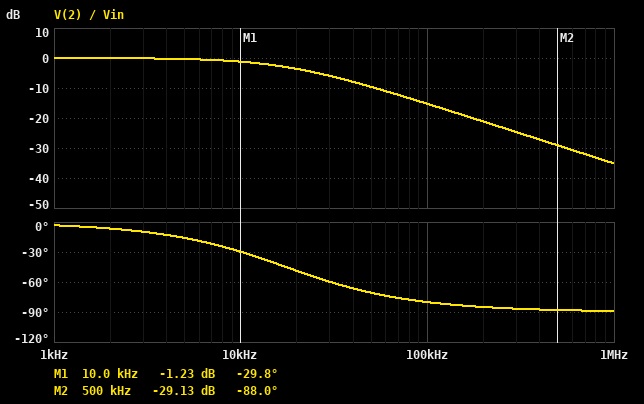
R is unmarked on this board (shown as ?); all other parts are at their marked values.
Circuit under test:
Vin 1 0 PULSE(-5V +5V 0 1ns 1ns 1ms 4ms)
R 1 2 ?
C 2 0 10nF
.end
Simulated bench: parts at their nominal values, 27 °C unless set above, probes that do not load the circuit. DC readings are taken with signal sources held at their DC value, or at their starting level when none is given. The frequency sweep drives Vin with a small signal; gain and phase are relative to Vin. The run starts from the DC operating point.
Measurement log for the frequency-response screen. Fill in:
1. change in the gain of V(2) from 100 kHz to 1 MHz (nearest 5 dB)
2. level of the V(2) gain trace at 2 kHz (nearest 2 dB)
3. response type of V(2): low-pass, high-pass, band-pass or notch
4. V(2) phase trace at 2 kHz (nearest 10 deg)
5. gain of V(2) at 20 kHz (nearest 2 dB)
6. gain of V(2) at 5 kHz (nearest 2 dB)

-20 dB
0 dB
low-pass
-10 deg
-4 dB
0 dB
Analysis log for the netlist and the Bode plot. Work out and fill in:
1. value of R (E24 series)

910 Ω
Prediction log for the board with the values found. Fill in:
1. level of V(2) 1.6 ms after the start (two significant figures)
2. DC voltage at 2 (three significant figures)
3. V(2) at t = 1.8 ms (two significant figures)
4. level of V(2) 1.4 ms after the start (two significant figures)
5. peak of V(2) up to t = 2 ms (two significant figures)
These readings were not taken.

-5.0 V
-5.00 V
-5.0 V
-5.0 V
5.0 V
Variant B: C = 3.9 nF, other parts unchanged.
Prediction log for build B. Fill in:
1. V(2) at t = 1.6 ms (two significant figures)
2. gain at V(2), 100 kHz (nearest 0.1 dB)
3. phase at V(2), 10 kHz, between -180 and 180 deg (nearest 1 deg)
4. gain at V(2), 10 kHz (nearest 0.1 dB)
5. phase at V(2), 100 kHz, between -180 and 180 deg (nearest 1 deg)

-5.0 V
-7.8 dB
-13 deg
-0.2 dB
-66 deg
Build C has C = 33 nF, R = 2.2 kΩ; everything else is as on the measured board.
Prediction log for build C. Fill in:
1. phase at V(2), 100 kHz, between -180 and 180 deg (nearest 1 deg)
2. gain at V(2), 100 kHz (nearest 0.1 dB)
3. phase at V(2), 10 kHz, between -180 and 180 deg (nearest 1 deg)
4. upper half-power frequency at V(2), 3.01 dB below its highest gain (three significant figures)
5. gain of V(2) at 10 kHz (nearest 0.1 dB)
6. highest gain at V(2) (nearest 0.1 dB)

-89 deg
-33.2 dB
-78 deg
2.19 kHz
-13.4 dB
0 dB
